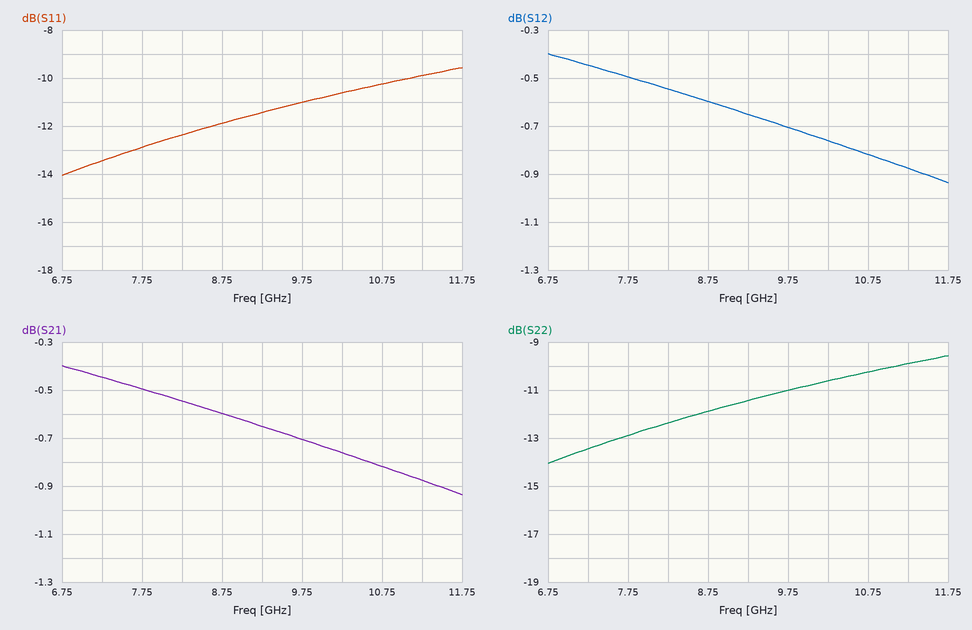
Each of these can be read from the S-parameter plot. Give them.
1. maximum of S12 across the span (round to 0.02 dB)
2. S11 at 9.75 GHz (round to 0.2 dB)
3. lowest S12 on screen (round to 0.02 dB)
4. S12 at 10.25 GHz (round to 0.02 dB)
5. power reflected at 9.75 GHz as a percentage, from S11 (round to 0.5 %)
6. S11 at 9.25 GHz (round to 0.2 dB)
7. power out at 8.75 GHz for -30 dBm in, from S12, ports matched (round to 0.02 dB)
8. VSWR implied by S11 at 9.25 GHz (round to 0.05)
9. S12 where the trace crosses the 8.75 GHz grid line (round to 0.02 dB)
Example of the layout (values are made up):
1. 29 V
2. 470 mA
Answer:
1. -0.40 dB
2. -11.0 dB
3. -0.94 dB
4. -0.76 dB
5. 8.0 %
6. -11.4 dB
7. -30.60 dBm
8. 1.75
9. -0.60 dB
